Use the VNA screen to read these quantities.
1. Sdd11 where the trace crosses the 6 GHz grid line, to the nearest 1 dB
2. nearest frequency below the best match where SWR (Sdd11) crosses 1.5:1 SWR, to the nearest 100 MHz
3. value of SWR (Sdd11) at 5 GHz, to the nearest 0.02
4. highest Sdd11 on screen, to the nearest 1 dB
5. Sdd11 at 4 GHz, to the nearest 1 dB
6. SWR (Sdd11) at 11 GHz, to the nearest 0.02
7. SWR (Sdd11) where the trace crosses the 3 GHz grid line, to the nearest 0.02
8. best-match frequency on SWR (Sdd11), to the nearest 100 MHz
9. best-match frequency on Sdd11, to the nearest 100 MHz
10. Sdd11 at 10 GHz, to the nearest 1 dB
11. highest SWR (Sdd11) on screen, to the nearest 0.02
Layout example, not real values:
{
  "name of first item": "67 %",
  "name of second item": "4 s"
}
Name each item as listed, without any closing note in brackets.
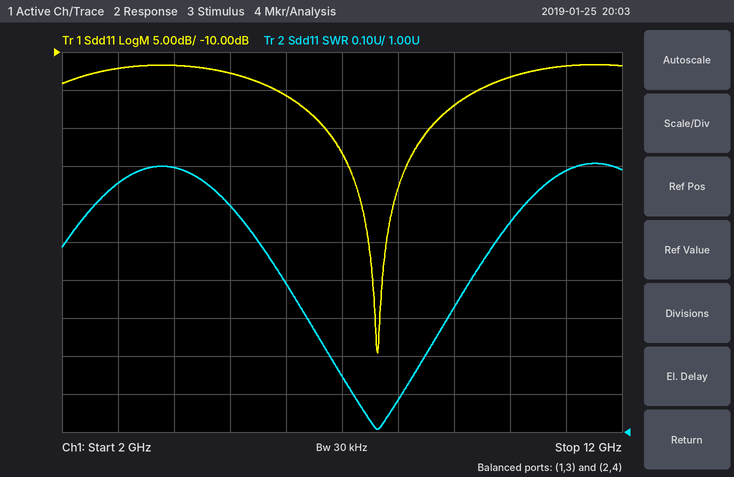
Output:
{
  "Sdd11 where the trace crosses the 6 GHz grid line, to the nearest 1 dB": "-16 dB",
  "nearest frequency below the best match where SWR (Sdd11) crosses 1.5:1 SWR, to the nearest 100 MHz": "5.5 GHz",
  "value of SWR (Sdd11) at 5 GHz, to the nearest 0.02": "1.60",
  "highest Sdd11 on screen, to the nearest 1 dB": "-12 dB",
  "Sdd11 at 4 GHz, to the nearest 1 dB": "-12 dB",
  "SWR (Sdd11) at 11 GHz, to the nearest 0.02": "1.68",
  "SWR (Sdd11) where the trace crosses the 3 GHz grid line, to the nearest 0.02": "1.66",
  "best-match frequency on SWR (Sdd11), to the nearest 100 MHz": "7.6 GHz",
  "best-match frequency on Sdd11, to the nearest 100 MHz": "7.6 GHz",
  "Sdd11 at 10 GHz, to the nearest 1 dB": "-13 dB",
  "highest SWR (Sdd11) on screen, to the nearest 0.02": "1.70"
}
